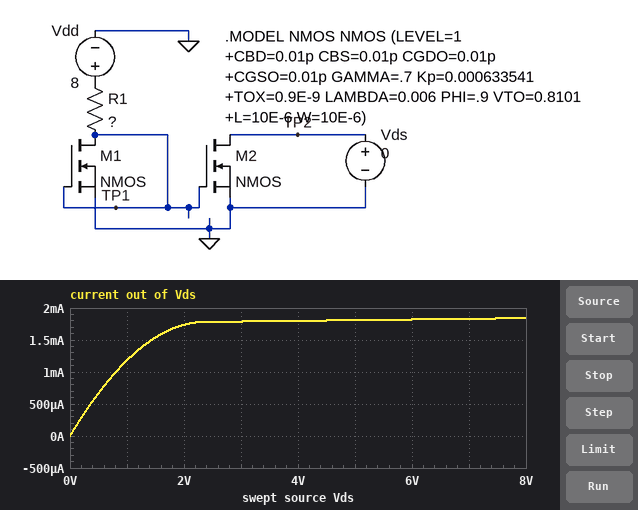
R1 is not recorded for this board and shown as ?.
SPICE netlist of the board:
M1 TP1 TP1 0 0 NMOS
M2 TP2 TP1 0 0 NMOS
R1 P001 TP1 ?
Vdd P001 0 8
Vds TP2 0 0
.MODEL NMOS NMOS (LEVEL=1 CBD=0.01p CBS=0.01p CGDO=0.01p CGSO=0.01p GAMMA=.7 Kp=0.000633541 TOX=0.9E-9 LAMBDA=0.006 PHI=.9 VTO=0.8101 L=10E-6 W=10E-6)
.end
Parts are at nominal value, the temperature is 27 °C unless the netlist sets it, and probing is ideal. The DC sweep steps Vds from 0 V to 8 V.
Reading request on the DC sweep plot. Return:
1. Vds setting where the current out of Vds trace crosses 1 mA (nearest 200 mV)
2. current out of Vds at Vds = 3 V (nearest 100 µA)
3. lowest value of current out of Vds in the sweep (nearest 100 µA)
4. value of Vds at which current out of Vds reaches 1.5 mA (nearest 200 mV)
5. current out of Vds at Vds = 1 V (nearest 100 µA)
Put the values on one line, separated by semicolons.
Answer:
800 mV; 1.8 mA; 0 A; 1.4 V; 1.2 mA
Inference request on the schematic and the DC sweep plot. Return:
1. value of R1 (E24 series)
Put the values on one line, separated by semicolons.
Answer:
2.7 kΩ
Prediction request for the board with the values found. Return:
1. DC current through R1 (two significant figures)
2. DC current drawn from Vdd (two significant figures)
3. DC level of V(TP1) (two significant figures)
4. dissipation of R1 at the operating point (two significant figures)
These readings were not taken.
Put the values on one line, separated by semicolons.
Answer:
1.8 mA; 1.8 mA; 3.2 V; 8.7 mW
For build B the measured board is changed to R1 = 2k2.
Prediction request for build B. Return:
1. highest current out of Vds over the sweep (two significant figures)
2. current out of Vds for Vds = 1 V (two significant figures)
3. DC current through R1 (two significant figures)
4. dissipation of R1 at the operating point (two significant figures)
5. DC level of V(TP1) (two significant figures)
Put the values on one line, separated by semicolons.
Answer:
2.2 mA; 1.3 mA; 2.1 mA; 9.8 mW; 3.4 V
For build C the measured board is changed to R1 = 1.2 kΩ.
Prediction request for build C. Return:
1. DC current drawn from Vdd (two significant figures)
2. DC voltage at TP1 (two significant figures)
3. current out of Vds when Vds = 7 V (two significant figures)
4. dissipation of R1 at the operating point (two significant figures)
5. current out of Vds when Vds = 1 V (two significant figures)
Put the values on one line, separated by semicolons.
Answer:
3.3 mA; 4.0 V; 3.4 mA; 13 mW; 1.7 mA
